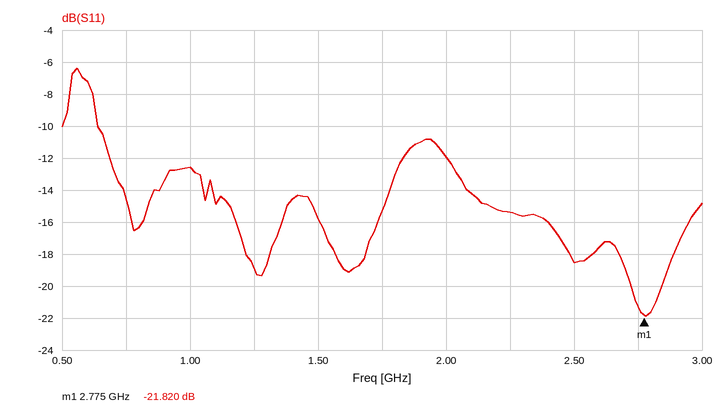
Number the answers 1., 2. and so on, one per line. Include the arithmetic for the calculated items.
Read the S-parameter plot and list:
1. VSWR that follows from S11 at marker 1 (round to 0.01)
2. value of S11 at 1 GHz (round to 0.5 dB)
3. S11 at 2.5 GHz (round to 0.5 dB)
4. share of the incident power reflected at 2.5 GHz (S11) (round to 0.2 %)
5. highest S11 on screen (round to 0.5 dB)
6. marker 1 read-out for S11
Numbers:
1. (1 + 0.0811)/(1 − 0.0811) ≈ 1.18
2. -12.5 dB
3. -18.5 dB
4. 10^(-18.5/10) ≈ 1.4 %
5. -6.5 dB
6. -21.820 dB
